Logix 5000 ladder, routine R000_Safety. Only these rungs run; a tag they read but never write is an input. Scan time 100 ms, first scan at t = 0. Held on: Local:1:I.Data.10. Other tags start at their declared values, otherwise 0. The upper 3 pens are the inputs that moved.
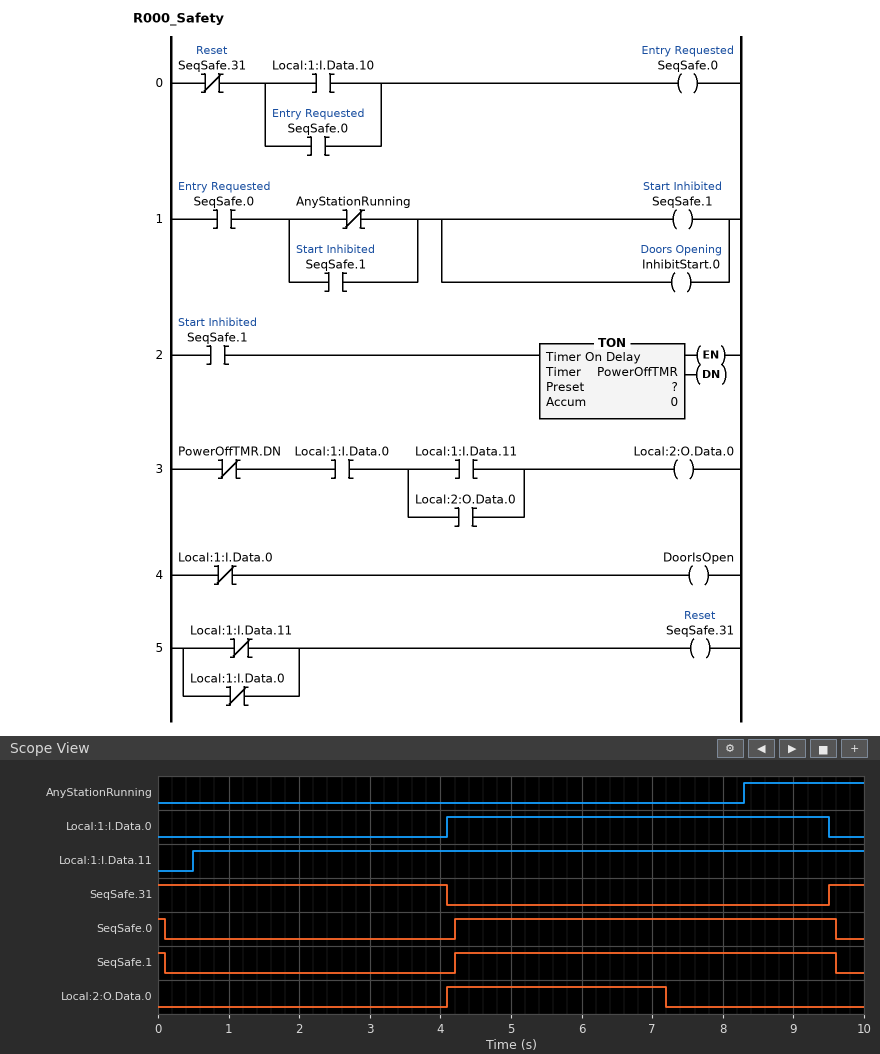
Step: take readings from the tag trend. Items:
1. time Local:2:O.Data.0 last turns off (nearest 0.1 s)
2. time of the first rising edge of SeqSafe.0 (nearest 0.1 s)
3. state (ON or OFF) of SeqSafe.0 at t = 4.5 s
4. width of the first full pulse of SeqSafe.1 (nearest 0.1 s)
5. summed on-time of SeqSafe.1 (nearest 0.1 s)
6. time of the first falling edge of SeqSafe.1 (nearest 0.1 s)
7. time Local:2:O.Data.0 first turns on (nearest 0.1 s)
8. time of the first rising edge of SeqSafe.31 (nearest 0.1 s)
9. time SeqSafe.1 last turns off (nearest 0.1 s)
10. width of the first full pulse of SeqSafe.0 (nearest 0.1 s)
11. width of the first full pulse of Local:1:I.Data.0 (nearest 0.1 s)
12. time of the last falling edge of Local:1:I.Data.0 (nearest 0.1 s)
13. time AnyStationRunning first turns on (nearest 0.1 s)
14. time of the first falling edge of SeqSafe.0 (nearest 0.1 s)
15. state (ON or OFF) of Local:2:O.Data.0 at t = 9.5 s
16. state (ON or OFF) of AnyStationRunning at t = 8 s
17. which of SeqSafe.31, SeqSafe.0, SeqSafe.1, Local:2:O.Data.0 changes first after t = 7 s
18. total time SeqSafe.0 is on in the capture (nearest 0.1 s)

7.2 s
4.2 s
ON
5.4 s
5.5 s
0.1 s
4.1 s
9.5 s
9.6 s
5.4 s
5.4 s
9.5 s
8.3 s
0.1 s
OFF
OFF
Local:2:O.Data.0
5.5 s
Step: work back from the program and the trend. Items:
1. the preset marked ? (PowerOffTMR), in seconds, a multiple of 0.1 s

3.0 s
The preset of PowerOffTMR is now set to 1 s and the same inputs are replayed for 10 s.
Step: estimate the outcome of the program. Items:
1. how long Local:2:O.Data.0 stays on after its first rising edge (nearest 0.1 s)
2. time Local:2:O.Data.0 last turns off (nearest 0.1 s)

1.1 s
5.2 s
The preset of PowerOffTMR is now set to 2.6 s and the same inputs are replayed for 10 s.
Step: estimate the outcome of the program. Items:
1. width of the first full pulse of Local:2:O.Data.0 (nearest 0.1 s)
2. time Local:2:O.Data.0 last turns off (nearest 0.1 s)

2.7 s
6.8 s
